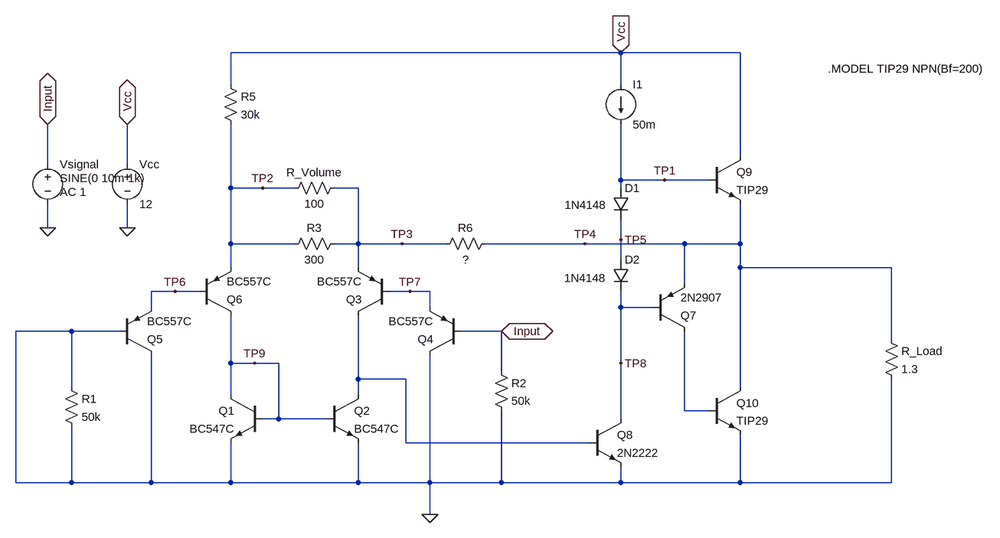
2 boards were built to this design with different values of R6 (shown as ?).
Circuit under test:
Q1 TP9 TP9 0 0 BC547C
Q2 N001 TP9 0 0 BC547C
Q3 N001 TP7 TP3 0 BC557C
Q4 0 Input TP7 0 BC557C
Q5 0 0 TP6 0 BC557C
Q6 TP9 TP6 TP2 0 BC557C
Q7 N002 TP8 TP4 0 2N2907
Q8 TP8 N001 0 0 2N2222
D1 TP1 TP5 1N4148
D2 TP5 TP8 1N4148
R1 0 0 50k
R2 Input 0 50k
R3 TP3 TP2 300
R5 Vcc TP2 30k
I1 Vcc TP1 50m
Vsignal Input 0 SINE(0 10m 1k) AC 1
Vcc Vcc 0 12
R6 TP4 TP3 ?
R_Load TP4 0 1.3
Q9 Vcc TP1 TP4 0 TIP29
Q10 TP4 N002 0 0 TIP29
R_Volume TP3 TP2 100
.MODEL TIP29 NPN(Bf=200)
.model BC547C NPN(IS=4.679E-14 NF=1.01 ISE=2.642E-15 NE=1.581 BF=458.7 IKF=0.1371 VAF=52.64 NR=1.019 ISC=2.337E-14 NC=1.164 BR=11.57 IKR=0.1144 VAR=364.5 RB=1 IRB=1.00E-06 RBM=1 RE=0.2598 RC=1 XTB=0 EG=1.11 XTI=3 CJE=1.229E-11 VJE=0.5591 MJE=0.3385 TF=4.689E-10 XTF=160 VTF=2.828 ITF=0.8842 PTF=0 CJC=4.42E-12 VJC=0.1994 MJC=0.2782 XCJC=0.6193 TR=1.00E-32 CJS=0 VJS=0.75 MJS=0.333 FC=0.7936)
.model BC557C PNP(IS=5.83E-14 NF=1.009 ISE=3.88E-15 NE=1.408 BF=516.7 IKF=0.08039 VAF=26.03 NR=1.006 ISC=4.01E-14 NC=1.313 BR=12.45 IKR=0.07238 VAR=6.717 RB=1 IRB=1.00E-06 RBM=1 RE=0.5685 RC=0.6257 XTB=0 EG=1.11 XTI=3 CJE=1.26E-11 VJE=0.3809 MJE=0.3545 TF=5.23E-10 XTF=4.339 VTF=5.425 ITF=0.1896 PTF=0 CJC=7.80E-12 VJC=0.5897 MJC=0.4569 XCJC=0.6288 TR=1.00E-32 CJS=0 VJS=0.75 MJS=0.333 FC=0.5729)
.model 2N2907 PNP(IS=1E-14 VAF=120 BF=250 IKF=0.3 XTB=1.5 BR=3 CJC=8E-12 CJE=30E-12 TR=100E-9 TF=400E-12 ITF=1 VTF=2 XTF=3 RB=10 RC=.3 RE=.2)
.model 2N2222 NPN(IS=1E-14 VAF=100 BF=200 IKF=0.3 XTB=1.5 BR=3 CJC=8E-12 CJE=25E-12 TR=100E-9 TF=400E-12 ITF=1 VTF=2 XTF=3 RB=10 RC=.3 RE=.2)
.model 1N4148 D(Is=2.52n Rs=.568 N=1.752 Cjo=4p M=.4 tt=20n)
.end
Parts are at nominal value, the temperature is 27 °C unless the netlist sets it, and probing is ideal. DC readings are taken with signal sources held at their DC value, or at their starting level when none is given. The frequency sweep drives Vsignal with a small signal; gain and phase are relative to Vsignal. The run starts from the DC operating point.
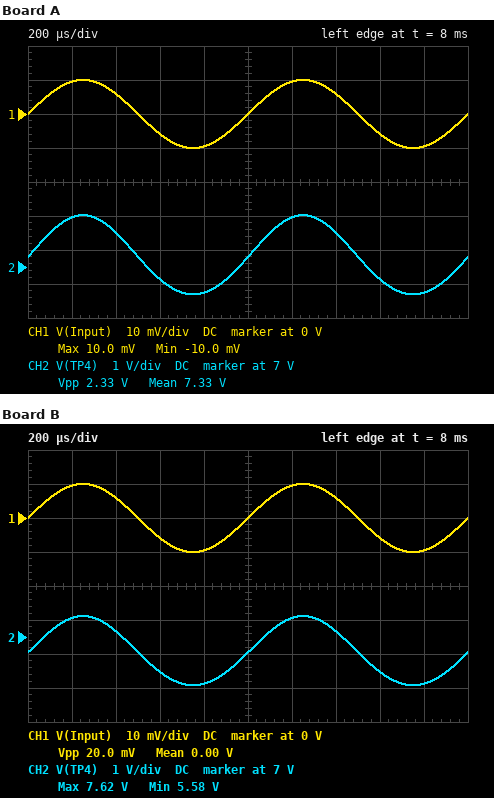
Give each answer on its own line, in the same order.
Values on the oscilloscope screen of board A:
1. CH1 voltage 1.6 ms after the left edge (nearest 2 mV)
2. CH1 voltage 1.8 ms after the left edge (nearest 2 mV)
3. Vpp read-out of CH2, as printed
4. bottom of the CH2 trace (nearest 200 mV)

-6 mV
-10 mV
2.33 V
6.2 V
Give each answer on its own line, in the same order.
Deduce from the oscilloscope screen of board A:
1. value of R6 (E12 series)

8.2 kΩ
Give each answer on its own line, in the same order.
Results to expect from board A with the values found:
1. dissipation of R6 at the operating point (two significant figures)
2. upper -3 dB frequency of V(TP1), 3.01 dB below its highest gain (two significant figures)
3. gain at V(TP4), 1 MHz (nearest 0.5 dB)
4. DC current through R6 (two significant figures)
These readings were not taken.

4.8 mW
230 kHz
35.0 dB
760 µA
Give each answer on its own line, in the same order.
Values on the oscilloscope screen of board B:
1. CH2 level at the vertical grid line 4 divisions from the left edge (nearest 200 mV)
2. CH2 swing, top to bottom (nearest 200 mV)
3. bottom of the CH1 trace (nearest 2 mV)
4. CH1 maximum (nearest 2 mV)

5.6 V
2.0 V
-10 mV
10 mV
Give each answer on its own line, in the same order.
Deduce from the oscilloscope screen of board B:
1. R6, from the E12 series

6.8 kΩ
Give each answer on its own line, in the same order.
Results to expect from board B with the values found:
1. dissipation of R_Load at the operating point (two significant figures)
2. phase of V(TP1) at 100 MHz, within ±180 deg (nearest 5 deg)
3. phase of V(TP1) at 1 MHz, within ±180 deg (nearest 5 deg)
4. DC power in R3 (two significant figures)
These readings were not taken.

33 W
-170 deg
-35 deg
470 nW
